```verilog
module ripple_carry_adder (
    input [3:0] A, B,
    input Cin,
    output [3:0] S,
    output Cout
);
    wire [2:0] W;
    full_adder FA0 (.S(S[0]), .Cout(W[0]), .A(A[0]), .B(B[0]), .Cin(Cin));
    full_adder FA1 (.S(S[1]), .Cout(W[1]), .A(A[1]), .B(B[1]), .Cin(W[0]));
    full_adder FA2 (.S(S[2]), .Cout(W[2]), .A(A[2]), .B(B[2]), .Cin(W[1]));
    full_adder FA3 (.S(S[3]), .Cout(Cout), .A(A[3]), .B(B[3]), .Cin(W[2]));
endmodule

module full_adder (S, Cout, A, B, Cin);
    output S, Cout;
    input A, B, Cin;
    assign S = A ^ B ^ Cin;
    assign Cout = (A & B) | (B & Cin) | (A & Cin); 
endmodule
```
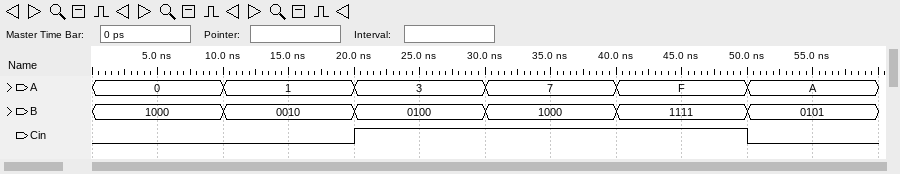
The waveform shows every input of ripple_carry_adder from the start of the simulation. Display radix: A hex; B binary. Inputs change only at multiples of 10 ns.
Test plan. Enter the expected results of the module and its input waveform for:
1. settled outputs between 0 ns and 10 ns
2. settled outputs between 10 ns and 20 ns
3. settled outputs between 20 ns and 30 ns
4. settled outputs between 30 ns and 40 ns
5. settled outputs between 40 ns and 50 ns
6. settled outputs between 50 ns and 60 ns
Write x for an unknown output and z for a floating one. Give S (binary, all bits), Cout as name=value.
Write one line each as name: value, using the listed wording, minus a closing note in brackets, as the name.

settled outputs between 0 ns and 10 ns: S=1000, Cout=0
settled outputs between 10 ns and 20 ns: S=0011, Cout=0
settled outputs between 20 ns and 30 ns: S=1000, Cout=0
settled outputs between 30 ns and 40 ns: S=0000, Cout=1
settled outputs between 40 ns and 50 ns: S=1111, Cout=1
settled outputs between 50 ns and 60 ns: S=1111, Cout=0
